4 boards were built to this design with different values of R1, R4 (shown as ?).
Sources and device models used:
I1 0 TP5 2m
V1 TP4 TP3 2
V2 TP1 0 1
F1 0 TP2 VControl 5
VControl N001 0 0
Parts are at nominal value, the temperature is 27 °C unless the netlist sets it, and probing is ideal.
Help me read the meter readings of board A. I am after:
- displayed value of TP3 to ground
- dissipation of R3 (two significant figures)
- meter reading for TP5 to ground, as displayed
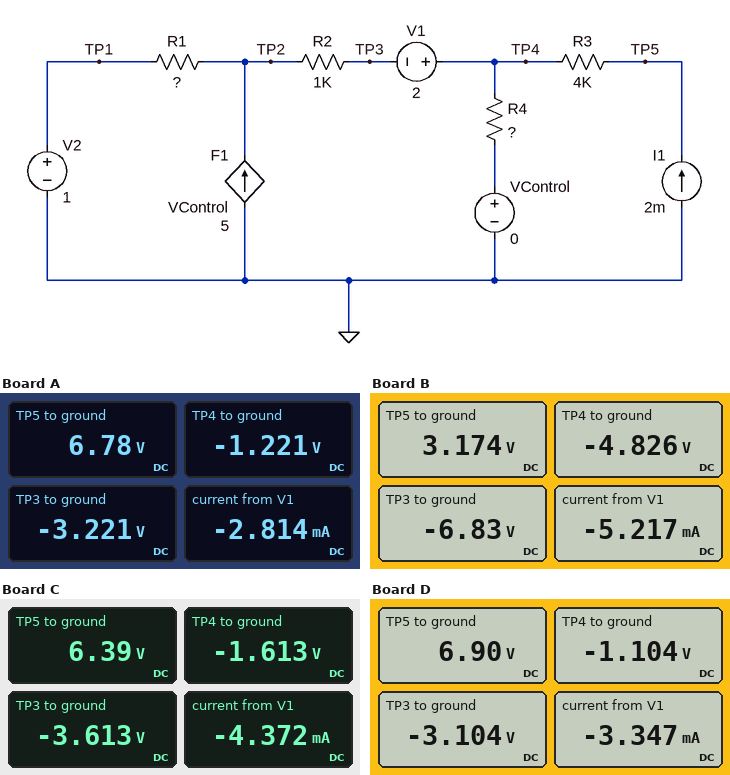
-3.221 V
16 mW
6.78 V
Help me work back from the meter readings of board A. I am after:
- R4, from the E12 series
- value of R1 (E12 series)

1.5 kΩ
5.6 kΩ
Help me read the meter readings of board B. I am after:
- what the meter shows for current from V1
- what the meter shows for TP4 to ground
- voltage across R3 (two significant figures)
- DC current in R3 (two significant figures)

-5.217 mA
-4.826 V
8.0 V
2.0 mA
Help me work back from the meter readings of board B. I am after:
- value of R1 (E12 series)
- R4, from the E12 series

1.2 kΩ
1.5 kΩ
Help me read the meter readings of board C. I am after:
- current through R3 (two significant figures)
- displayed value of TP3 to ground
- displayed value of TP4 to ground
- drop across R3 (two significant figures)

2.0 mA
-3.613 V
-1.613 V
8.0 V
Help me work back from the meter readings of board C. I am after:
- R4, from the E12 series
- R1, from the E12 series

680 Ω
1.2 kΩ
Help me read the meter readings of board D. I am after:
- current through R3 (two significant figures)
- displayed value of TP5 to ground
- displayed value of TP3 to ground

2.0 mA
6.90 V
-3.104 V
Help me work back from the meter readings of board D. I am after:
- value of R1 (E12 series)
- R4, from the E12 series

2.2 kΩ
820 Ω
